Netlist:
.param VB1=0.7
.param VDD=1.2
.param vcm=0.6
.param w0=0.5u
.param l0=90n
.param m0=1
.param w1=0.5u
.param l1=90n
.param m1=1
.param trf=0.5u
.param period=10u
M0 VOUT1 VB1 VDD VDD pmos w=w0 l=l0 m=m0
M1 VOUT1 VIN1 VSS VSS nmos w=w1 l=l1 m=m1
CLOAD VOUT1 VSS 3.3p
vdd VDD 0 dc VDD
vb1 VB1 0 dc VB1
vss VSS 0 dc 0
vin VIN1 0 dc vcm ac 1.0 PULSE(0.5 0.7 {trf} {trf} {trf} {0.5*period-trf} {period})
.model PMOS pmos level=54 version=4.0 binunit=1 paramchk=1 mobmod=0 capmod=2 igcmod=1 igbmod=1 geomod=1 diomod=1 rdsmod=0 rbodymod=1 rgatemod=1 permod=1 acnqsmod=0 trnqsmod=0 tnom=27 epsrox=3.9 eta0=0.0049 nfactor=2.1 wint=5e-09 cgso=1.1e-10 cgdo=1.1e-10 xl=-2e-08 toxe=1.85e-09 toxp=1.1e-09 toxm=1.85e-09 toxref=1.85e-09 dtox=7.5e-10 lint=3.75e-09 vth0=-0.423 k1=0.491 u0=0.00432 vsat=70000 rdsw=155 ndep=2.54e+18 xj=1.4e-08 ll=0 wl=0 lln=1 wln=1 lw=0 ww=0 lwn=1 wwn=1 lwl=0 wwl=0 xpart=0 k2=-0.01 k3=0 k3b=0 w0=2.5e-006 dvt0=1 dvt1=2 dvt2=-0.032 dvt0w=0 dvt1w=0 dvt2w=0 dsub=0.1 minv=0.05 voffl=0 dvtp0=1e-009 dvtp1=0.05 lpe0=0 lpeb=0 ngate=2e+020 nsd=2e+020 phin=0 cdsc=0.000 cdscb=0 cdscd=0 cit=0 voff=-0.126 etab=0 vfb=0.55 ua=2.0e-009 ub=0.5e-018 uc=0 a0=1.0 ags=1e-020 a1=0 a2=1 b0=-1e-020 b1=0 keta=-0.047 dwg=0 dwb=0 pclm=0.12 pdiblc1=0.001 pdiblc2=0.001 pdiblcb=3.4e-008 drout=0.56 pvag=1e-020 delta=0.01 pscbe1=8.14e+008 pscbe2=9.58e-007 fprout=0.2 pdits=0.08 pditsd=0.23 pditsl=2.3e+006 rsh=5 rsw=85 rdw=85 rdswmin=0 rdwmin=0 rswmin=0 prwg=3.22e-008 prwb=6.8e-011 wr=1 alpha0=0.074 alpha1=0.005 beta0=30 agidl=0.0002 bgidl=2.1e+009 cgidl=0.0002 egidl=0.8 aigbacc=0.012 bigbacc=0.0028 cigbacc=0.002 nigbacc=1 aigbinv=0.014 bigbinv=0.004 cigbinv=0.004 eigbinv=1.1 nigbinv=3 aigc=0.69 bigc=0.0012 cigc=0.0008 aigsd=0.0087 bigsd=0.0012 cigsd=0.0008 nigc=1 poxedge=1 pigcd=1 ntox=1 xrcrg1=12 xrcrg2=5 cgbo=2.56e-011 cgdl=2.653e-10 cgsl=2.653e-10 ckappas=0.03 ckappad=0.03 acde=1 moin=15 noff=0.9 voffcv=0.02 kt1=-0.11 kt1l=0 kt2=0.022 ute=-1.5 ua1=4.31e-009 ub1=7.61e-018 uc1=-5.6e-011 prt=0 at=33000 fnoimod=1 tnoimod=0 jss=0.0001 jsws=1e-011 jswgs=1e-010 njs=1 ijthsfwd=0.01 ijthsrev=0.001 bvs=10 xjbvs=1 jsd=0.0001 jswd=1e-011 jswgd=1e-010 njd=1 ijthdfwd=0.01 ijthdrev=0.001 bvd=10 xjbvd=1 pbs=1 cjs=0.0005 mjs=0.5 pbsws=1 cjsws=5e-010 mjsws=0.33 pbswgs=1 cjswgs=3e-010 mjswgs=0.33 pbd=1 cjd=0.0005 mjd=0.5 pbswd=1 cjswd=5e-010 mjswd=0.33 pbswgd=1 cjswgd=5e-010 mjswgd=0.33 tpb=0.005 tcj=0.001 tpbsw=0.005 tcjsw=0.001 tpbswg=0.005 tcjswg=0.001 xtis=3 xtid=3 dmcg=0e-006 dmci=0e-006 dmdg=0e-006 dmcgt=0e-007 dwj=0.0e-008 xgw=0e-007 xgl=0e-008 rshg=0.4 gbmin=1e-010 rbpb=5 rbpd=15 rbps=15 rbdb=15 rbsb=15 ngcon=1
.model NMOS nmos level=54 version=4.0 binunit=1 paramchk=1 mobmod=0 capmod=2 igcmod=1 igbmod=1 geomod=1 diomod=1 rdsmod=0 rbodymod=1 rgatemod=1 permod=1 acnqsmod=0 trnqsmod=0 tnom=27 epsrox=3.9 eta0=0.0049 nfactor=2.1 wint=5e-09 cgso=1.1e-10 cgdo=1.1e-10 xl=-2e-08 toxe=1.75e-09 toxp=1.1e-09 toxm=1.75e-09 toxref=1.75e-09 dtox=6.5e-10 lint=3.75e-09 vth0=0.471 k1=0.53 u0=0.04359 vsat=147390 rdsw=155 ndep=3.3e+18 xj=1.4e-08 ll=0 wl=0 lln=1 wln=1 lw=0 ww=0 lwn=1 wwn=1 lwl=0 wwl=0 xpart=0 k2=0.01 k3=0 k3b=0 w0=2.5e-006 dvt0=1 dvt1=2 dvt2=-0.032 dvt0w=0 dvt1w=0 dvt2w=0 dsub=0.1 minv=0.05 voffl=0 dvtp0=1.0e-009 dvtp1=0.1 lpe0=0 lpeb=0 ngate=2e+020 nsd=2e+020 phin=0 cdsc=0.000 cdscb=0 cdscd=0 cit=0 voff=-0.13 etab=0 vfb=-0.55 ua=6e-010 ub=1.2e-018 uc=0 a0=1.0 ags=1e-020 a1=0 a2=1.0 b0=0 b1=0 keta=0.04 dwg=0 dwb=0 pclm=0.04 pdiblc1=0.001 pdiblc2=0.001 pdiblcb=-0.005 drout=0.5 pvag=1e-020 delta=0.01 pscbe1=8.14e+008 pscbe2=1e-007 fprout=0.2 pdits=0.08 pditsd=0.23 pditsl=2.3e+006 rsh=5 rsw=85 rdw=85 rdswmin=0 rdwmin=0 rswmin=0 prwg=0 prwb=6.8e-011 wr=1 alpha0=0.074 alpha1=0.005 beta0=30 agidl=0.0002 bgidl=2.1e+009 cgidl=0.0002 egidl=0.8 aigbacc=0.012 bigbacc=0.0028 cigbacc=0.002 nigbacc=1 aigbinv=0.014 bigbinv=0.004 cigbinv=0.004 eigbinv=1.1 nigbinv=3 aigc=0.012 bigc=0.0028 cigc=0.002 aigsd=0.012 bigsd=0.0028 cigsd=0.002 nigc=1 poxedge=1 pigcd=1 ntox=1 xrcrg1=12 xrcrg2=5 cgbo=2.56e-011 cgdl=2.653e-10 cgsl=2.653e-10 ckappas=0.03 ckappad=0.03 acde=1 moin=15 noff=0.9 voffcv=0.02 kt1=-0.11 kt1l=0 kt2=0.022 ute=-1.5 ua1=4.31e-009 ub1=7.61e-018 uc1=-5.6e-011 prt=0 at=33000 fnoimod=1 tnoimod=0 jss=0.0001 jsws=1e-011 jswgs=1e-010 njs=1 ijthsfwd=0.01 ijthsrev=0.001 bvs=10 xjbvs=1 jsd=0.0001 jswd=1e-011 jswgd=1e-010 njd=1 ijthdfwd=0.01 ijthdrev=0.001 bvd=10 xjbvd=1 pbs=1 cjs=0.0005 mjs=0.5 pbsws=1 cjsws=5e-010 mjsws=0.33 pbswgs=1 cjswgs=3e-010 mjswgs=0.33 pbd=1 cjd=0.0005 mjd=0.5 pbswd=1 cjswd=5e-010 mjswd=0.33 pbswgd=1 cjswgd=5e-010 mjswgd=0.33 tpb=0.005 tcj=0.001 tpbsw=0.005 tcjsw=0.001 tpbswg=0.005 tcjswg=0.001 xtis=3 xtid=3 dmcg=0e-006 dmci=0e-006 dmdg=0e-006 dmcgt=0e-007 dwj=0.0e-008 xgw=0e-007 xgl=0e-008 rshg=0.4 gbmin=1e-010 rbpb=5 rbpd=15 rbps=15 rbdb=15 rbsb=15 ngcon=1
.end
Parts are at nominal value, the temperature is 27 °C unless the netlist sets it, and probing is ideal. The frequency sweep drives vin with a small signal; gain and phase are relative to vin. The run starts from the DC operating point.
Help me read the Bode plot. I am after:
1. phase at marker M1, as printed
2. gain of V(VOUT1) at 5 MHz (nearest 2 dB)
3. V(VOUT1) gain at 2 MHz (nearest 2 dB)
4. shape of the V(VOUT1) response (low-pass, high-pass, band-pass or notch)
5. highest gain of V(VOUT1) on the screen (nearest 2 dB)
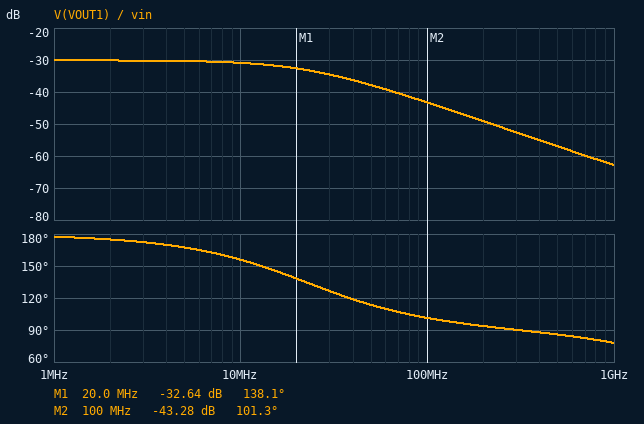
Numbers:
138.1 deg
-30 dB
-30 dB
low-pass
-30 dB
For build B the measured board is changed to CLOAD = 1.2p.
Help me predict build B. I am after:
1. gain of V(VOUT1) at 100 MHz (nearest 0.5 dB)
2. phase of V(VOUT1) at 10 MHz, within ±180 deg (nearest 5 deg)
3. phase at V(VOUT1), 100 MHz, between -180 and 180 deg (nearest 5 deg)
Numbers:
-35.5 dB
170 deg
120 deg
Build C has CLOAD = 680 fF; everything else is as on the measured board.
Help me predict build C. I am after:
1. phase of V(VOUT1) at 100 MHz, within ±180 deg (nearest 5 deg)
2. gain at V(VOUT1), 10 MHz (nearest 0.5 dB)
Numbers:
135 deg
-30.0 dB
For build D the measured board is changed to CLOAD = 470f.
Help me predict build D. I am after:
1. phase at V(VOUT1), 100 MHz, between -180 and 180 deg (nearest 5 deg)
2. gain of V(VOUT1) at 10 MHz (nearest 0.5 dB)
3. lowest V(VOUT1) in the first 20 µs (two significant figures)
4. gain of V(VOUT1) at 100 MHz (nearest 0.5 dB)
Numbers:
145 deg
-30.0 dB
3.4 mV
-31.5 dB
